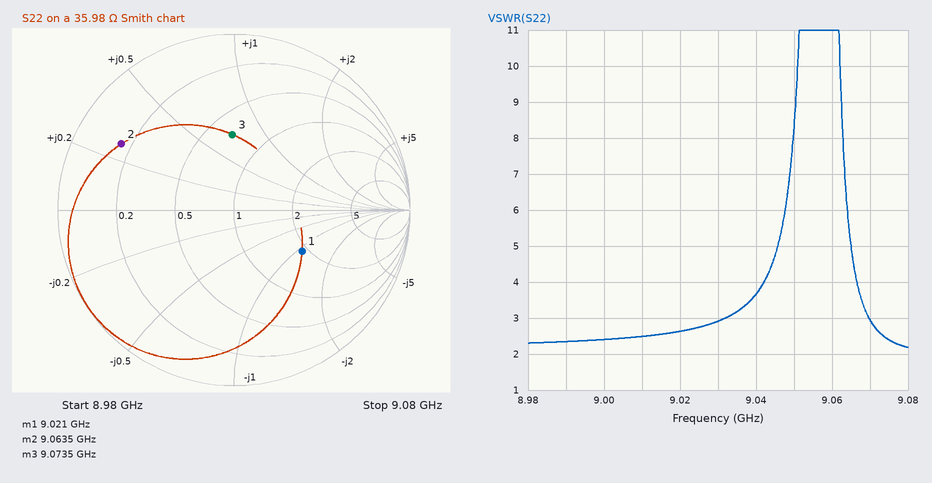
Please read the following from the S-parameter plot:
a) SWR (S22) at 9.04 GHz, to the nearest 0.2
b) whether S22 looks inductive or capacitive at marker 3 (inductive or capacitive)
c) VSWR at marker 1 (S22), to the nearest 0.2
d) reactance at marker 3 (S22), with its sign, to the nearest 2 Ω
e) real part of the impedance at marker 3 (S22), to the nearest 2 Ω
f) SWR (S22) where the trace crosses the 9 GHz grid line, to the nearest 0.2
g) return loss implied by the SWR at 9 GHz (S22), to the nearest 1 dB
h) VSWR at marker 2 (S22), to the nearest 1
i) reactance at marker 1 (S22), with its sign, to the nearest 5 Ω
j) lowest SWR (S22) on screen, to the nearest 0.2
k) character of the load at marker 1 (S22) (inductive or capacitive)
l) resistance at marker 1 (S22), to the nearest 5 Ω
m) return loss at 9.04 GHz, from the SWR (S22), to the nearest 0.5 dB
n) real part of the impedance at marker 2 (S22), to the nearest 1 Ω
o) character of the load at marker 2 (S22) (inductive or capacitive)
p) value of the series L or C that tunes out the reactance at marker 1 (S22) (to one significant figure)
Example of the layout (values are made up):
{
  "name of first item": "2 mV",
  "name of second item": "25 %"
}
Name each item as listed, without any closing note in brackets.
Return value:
{
  "SWR (S22) at 9.04 GHz, to the nearest 0.2": "3.6",
  "whether S22 looks inductive or capacitive at marker 3": "inductive",
  "VSWR at marker 1 (S22), to the nearest 0.2": "2.6",
  "reactance at marker 3 (S22), with its sign, to the nearest 2 Ω": "+26 Ω",
  "real part of the impedance at marker 3 (S22), to the nearest 2 Ω": "24 Ω",
  "SWR (S22) where the trace crosses the 9 GHz grid line, to the nearest 0.2": "2.4",
  "return loss implied by the SWR at 9 GHz (S22), to the nearest 1 dB": "8 dB",
  "VSWR at marker 2 (S22), to the nearest 1": "7",
  "reactance at marker 1 (S22), with its sign, to the nearest 5 Ω": "-40 Ω",
  "lowest SWR (S22) on screen, to the nearest 0.2": "2.2",
  "character of the load at marker 1 (S22)": "capacitive",
  "resistance at marker 1 (S22), to the nearest 5 Ω": "65 Ω",
  "return loss at 9.04 GHz, from the SWR (S22), to the nearest 0.5 dB": "5.0 dB",
  "real part of the impedance at marker 2 (S22), to the nearest 1 Ω": "6 Ω",
  "character of the load at marker 2 (S22)": "inductive",
  "value of the series L or C that tunes out the reactance at marker 1 (S22)": "700 pH"
}
